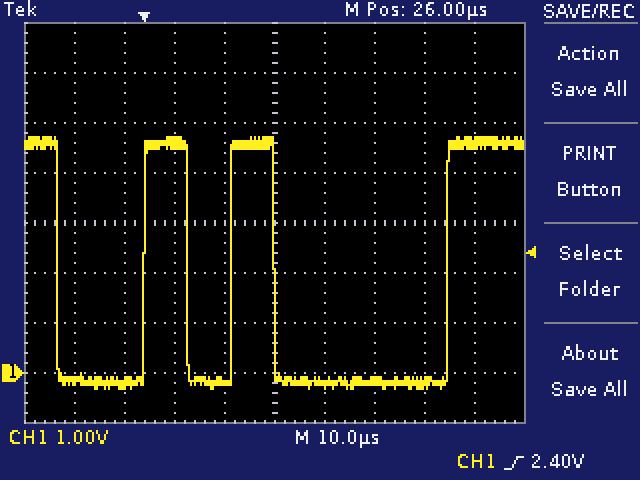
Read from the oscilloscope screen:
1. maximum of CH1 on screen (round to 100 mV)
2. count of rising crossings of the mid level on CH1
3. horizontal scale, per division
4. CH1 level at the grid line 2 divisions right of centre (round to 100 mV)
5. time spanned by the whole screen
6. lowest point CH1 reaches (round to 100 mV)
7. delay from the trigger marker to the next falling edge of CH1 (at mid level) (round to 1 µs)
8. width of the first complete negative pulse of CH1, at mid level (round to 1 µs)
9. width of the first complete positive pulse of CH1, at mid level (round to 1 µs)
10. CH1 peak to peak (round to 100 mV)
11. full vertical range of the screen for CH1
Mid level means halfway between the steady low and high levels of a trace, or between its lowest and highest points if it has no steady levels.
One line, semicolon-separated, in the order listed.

4.7 V; 3; 10 µs; -200 mV; 100 µs; -300 mV; 9 µs; 17 µs; 9 µs; 5.0 V; 8 V
